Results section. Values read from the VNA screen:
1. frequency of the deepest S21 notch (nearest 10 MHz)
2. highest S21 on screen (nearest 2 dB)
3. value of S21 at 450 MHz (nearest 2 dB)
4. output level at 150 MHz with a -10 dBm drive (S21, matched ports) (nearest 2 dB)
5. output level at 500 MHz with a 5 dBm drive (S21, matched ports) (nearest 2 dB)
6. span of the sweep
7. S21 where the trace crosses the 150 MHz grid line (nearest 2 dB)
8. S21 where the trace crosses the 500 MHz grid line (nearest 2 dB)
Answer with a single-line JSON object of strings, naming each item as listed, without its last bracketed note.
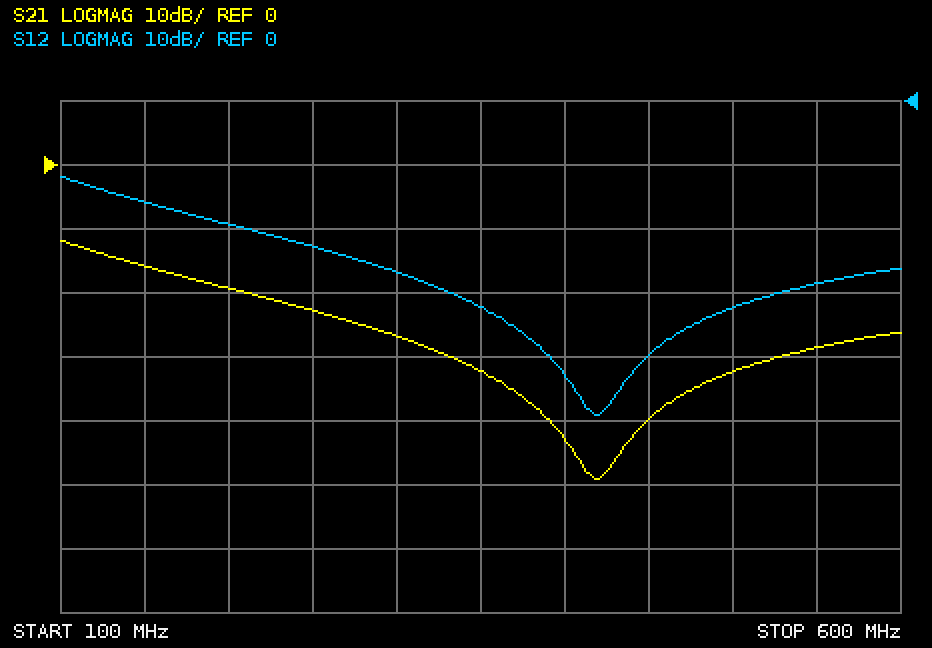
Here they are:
{"frequency of the deepest S21 notch": "420 MHz", "highest S21 on screen": "-12 dB", "value of S21 at 450 MHz": "-40 dB", "output level at 150 MHz with a -10 dBm drive (S21, matched ports)": "-26 dBm", "output level at 500 MHz with a 5 dBm drive (S21, matched ports)": "-28 dBm", "span of the sweep": "500 MHz", "S21 where the trace crosses the 150 MHz grid line": "-16 dB", "S21 where the trace crosses the 500 MHz grid line": "-32 dB"}
